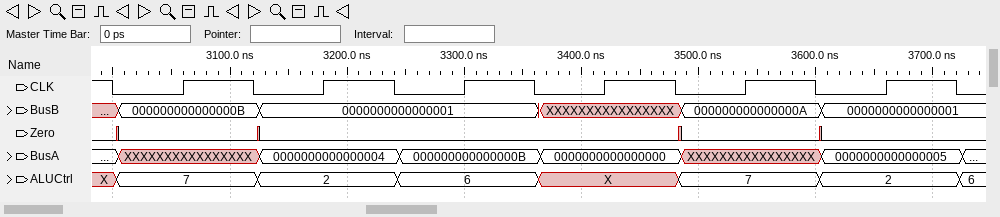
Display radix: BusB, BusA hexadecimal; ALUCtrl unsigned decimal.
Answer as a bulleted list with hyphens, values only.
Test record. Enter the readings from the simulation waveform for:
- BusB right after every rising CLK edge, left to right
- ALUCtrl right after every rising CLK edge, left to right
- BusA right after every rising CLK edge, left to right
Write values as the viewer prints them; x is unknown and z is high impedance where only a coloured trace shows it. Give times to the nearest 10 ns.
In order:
- 000000000000000B, 0000000000000001, 0000000000000001, XXXXXXXXXXXXXXXX, 000000000000000A, 0000000000000001
- 7, 2, 6, X, 7, 2
- XXXXXXXXXXXXXXXX, 0000000000000004, 000000000000000B, 0000000000000000, XXXXXXXXXXXXXXXX, 0000000000000005
